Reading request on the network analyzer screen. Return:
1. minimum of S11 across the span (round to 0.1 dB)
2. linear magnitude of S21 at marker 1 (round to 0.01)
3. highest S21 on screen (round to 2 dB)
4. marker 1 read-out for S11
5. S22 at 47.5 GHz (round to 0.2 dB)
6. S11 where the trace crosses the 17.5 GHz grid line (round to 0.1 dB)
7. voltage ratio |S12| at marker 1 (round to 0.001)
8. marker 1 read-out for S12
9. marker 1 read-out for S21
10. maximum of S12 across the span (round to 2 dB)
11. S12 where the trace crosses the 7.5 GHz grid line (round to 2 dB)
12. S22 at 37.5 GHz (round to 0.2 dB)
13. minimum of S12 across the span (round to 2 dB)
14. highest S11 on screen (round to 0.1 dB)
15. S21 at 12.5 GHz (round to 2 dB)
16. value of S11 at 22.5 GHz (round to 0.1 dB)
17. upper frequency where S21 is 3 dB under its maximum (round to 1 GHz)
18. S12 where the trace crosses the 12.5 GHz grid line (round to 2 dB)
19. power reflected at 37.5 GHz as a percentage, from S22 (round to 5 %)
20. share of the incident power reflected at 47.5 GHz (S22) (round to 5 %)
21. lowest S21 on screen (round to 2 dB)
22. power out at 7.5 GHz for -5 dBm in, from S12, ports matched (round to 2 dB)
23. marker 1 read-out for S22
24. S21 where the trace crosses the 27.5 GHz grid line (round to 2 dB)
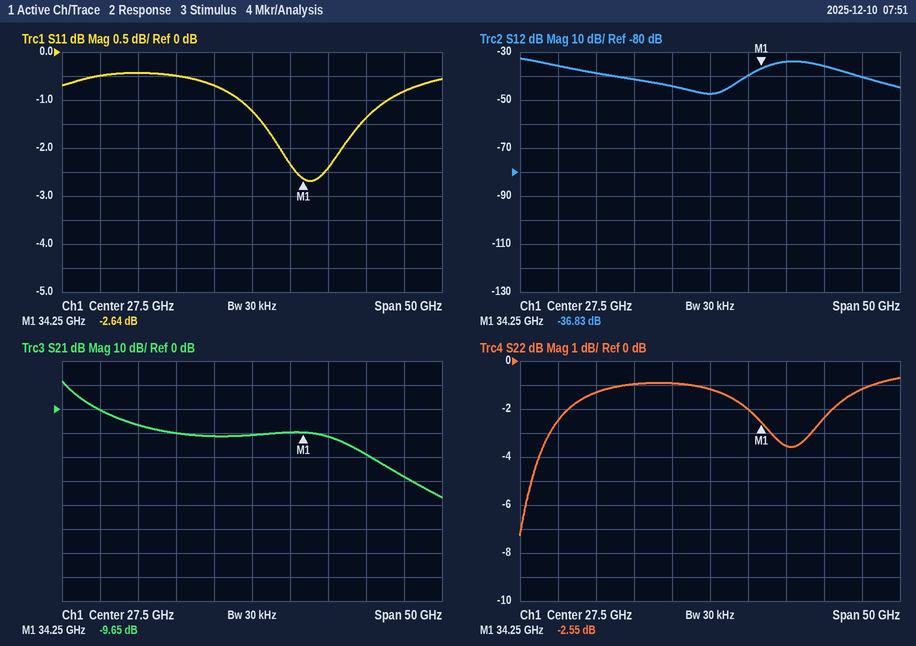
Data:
-2.7 dB
0.33
12 dB
-2.64 dB
-1.2 dB
-0.5 dB
0.014
-36.83 dB
-9.65 dB
-32 dB
-36 dB
-3.6 dB
-48 dB
-0.4 dB
-6 dB
-0.7 dB
3 GHz
-38 dB
45 %
75 %
-36 dB
-40 dBm
-2.55 dB
-10 dB
